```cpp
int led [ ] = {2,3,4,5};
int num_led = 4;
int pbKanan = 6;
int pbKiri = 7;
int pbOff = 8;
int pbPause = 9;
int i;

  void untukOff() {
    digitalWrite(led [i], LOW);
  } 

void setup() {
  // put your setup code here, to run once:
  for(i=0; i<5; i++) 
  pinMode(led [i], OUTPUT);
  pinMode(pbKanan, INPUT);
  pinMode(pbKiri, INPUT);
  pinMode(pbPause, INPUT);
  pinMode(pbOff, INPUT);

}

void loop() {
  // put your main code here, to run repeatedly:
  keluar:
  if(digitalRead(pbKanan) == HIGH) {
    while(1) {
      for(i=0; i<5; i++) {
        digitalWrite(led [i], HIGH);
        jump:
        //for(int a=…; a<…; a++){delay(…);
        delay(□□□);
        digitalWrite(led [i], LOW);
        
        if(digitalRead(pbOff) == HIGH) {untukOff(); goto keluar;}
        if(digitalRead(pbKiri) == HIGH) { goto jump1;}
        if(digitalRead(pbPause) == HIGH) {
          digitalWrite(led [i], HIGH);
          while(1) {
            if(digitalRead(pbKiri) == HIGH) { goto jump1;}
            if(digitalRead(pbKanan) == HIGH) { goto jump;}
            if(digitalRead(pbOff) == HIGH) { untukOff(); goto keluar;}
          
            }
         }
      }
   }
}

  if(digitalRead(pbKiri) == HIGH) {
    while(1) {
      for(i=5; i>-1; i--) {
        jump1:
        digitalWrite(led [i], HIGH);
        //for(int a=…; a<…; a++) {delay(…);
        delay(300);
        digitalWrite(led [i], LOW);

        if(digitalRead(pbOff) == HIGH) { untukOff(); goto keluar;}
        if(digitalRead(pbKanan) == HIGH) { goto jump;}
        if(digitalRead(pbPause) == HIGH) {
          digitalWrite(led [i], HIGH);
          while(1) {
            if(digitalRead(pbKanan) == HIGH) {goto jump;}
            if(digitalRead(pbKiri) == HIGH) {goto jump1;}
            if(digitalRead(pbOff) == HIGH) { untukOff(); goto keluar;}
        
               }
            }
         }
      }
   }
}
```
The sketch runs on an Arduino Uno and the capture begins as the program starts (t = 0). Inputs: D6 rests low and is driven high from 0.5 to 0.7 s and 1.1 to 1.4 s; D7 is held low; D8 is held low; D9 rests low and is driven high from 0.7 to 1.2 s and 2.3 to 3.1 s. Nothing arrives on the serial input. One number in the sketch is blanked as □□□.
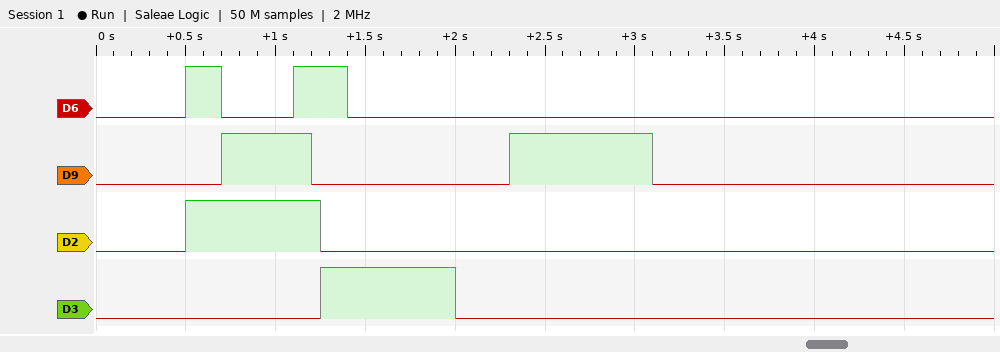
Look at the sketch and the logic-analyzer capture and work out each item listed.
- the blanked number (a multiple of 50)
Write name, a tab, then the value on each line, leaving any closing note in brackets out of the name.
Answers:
the blanked number	750
